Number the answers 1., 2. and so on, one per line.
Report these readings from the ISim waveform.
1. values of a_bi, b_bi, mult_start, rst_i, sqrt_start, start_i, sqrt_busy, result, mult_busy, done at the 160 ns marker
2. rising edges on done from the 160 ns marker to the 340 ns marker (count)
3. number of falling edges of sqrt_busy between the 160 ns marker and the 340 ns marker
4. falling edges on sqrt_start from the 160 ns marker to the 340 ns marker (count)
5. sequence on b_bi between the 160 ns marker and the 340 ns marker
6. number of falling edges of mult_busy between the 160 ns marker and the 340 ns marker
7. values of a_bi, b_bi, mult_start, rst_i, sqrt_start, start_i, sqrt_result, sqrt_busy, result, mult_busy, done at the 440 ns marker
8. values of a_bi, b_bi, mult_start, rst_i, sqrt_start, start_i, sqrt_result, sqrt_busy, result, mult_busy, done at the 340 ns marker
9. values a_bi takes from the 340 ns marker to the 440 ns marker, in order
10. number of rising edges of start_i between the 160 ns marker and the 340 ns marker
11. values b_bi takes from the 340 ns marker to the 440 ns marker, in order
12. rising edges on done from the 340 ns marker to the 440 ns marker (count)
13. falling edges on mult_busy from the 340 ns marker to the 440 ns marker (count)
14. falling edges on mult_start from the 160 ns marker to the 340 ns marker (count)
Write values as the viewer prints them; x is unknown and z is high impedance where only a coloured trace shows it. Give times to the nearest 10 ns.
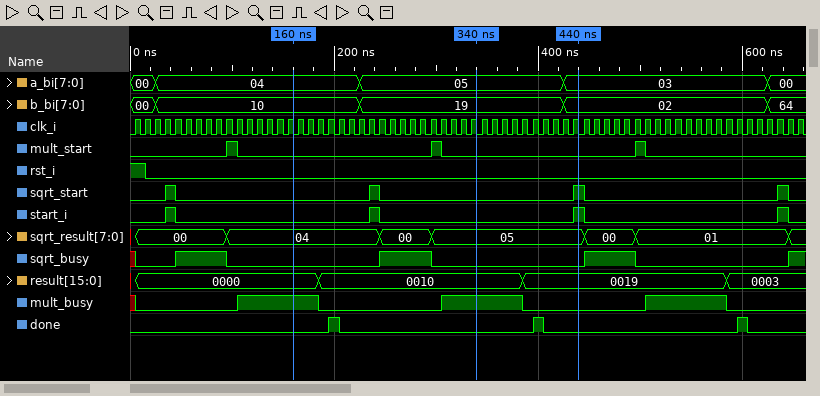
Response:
1. a_bi=04, b_bi=10, mult_start=0, rst_i=0, sqrt_start=0, start_i=0, sqrt_busy=0, result=0000, mult_busy=1, done=0
2. 1
3. 1
4. 1
5. 10, 19
6. 1
7. a_bi=03, b_bi=02, mult_start=0, rst_i=0, sqrt_start=1, start_i=1, sqrt_result=05, sqrt_busy=0, result=0019, mult_busy=0, done=0
8. a_bi=05, b_bi=19, mult_start=0, rst_i=0, sqrt_start=0, start_i=0, sqrt_result=05, sqrt_busy=0, result=0010, mult_busy=1, done=0
9. 05, 03
10. 1
11. 19, 02
12. 1
13. 1
14. 1
